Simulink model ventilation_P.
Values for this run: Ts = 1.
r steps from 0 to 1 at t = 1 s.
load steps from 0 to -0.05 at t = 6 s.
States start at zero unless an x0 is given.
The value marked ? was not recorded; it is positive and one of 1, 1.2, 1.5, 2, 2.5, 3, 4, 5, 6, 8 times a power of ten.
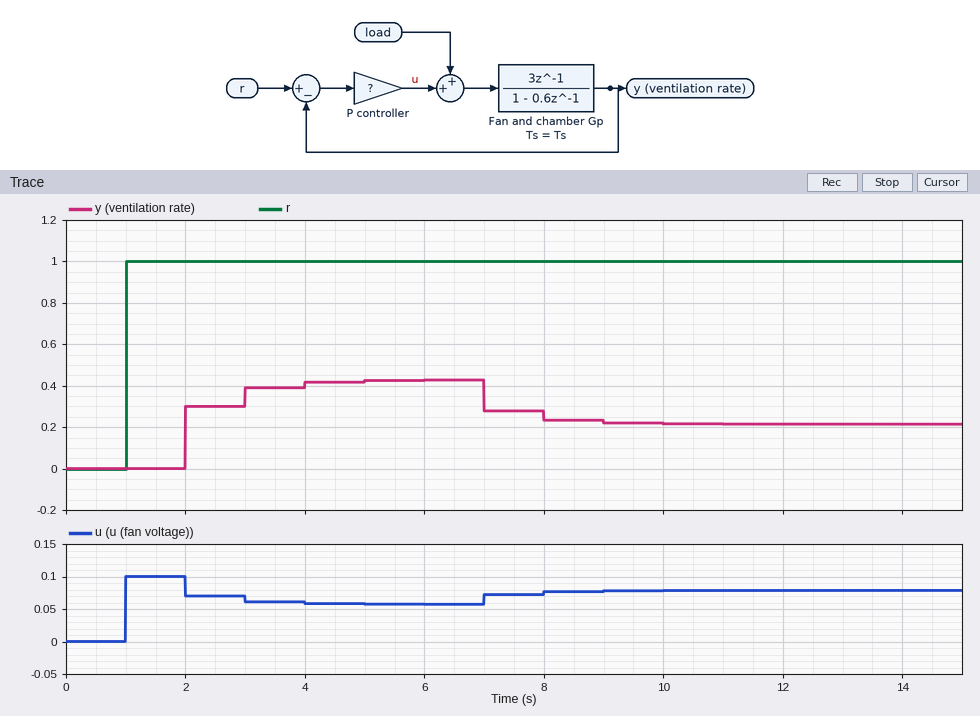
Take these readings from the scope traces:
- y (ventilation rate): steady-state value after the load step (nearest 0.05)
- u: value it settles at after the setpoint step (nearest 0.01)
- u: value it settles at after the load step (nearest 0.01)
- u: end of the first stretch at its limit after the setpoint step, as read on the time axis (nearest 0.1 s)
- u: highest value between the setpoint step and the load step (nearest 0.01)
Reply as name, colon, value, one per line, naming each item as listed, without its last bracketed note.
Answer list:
y (ventilation rate): steady-state value after the load step: 0.20
u: value it settles at after the setpoint step: 0.06
u: value it settles at after the load step: 0.08
u: end of the first stretch at its limit after the setpoint step, as read on the time axis: 2.0 s
u: highest value between the setpoint step and the load step: 0.10
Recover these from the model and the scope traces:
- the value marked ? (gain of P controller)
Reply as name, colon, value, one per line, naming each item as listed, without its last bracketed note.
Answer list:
the value marked ?: 0.1
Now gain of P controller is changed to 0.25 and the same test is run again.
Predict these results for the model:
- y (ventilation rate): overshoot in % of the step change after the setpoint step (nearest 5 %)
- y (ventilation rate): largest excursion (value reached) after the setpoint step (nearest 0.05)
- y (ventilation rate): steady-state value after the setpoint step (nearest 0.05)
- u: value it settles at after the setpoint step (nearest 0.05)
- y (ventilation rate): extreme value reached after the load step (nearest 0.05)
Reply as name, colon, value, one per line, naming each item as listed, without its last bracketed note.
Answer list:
y (ventilation rate): overshoot in % of the step change after the setpoint step: 15 %
y (ventilation rate): largest excursion (value reached) after the setpoint step: 0.75
y (ventilation rate): steady-state value after the setpoint step: 0.65
u: value it settles at after the setpoint step: 0.10
y (ventilation rate): extreme value reached after the load step: 0.50
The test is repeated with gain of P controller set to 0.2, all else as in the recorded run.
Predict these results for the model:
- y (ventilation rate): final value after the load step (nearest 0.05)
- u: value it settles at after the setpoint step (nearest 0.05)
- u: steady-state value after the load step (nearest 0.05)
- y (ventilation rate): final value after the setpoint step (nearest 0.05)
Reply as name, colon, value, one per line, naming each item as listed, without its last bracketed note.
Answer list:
y (ventilation rate): final value after the load step: 0.45
u: value it settles at after the setpoint step: 0.10
u: steady-state value after the load step: 0.10
y (ventilation rate): final value after the setpoint step: 0.60
